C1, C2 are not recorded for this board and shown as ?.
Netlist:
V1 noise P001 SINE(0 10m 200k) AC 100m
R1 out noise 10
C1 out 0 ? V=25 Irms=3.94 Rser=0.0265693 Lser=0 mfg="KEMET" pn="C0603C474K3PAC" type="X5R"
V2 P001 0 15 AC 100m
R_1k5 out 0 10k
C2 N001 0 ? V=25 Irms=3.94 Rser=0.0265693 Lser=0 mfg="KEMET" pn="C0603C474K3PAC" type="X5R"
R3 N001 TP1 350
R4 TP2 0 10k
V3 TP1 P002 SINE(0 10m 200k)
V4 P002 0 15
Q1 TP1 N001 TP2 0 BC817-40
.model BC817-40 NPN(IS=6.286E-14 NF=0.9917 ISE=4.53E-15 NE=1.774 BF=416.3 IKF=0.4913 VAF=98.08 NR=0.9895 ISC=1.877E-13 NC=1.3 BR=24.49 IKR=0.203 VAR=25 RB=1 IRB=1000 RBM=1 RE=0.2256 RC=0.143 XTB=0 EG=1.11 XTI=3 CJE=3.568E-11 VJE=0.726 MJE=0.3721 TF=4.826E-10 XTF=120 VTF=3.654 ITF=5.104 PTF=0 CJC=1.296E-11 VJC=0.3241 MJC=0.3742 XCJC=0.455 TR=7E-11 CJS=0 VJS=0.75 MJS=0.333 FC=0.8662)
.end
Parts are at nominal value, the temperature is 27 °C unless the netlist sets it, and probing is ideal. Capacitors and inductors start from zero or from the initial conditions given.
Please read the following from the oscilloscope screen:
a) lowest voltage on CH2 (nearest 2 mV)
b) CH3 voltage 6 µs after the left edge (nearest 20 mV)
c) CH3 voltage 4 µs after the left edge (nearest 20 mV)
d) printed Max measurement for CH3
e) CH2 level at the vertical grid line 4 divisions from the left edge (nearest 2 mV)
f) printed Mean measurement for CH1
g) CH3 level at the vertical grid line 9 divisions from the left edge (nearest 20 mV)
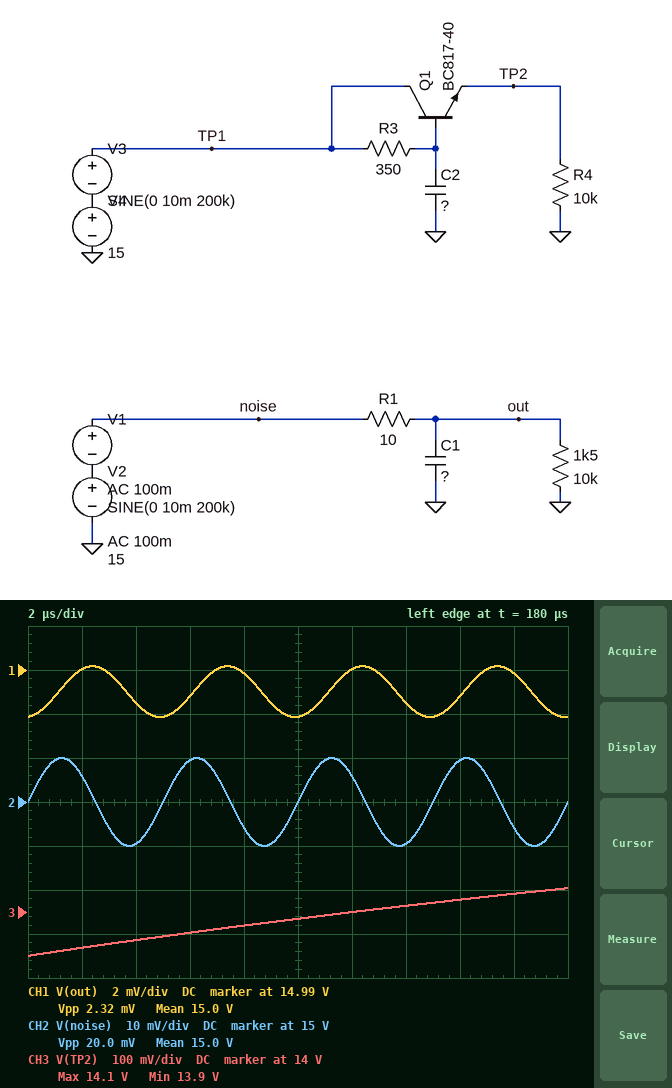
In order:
14.990 V
13.96 V
13.94 V
14.1 V
14.994 V
15.0 V
14.04 V
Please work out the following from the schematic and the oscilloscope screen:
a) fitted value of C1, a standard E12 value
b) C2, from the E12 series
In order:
680 nF
150 nF
